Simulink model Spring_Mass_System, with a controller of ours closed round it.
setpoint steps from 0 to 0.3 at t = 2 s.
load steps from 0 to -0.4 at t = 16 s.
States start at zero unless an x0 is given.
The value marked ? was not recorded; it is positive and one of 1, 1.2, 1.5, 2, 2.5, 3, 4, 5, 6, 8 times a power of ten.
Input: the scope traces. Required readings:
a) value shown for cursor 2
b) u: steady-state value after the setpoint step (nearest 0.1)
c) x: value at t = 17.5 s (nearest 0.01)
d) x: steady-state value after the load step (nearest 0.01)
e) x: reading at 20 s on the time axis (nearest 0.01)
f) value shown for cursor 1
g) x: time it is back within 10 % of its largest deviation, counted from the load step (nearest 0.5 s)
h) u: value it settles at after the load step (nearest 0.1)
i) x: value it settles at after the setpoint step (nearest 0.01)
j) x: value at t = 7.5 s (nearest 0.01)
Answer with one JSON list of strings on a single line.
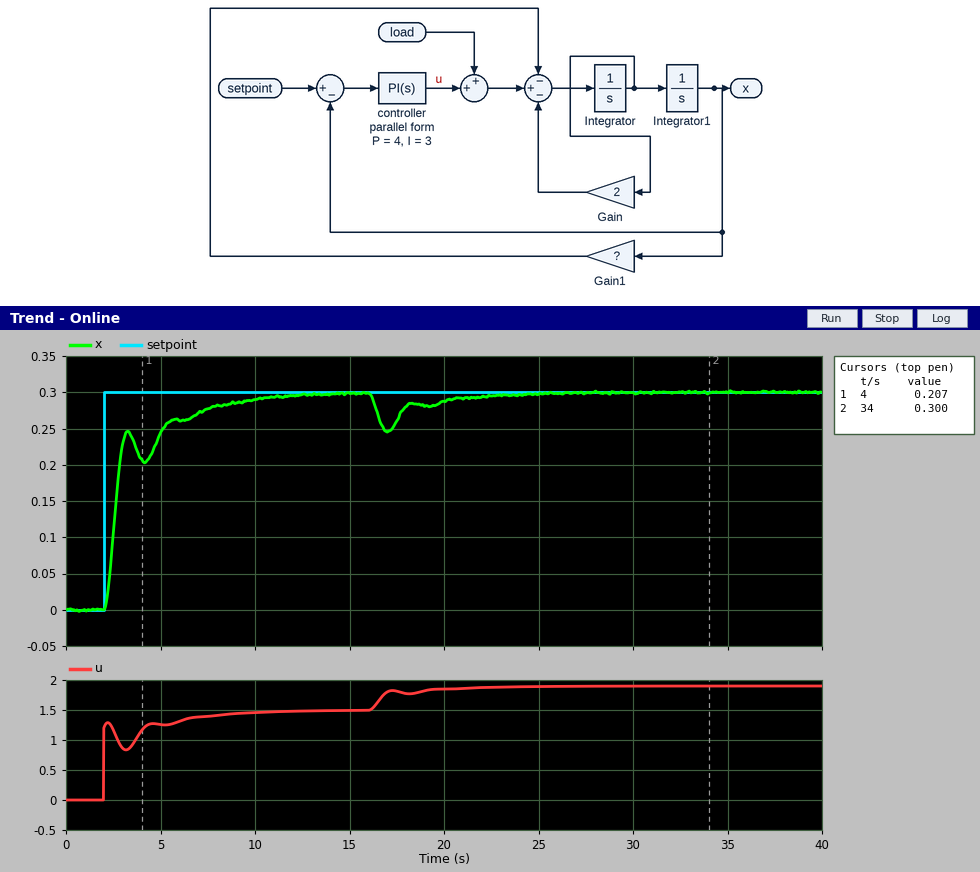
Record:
["0.300", "1.5", "0.26", "0.30", "0.29", "0.207", "6.5 s", "1.9", "0.30", "0.28"]
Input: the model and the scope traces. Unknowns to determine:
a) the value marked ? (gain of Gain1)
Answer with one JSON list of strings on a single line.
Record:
["5"]
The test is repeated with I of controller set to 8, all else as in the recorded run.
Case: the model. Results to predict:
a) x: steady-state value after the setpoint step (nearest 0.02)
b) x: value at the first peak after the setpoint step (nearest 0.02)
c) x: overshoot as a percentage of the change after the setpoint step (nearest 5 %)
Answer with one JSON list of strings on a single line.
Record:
["0.30", "0.34", "15 %"]
